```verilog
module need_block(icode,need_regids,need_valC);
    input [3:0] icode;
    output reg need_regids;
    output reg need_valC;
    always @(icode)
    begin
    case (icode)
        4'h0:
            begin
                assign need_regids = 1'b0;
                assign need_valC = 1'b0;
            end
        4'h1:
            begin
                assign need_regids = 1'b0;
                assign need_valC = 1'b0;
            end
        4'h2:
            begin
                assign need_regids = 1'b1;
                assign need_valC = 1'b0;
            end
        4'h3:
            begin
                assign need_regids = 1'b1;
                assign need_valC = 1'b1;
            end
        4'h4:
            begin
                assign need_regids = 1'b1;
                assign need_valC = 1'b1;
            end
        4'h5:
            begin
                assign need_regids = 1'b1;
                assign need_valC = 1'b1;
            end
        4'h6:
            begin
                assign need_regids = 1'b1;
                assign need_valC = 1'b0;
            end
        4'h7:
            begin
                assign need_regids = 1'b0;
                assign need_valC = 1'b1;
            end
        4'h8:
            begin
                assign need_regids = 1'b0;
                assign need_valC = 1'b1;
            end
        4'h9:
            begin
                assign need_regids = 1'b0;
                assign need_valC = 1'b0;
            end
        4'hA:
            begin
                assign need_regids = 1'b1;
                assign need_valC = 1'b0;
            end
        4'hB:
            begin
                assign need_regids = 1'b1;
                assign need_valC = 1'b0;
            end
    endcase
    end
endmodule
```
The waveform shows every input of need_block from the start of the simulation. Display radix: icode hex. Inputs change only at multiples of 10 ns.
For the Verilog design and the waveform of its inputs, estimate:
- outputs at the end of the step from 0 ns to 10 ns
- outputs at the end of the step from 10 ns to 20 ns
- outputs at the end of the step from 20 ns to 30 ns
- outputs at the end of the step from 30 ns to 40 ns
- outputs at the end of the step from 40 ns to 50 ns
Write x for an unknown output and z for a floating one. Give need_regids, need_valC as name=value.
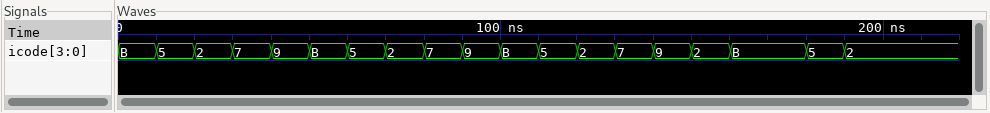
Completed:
need_regids=1, need_valC=0
need_regids=1, need_valC=1
need_regids=1, need_valC=0
need_regids=0, need_valC=1
need_regids=0, need_valC=0
